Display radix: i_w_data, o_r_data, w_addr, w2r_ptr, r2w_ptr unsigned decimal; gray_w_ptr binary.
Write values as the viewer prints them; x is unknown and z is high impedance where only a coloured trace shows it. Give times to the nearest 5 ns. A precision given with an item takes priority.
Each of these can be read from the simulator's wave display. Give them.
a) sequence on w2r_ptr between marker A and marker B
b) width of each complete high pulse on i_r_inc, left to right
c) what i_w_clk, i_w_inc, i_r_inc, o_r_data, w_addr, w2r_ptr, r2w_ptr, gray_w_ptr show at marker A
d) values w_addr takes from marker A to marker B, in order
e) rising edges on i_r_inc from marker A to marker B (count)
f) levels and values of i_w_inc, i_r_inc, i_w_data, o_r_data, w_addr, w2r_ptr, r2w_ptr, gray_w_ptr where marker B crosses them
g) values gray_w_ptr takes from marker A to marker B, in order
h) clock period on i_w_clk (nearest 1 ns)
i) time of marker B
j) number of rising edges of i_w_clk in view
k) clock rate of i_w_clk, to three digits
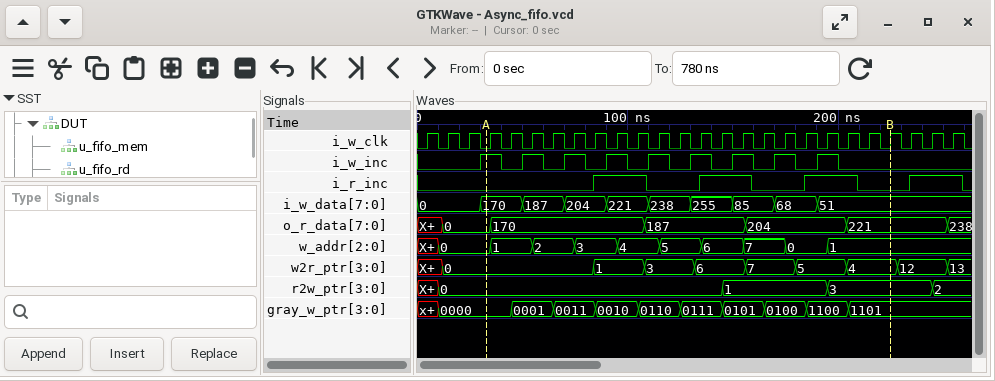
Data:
0, 1, 3, 6, 7, 5, 4
25 ns, 25 ns, 25 ns, 25 ns
i_w_clk=0, i_w_inc=1, i_r_inc=0, o_r_data=0, w_addr=0, w2r_ptr=0, r2w_ptr=0, gray_w_ptr=0000
0, 1, 2, 3, 4, 5, 6, 7, 0, 1
3
i_w_inc=0, i_r_inc=0, i_w_data=51, o_r_data=221, w_addr=1, w2r_ptr=4, r2w_ptr=3, gray_w_ptr=1101
0000, 0001, 0011, 0010, 0110, 0111, 0101, 0100, 1100, 1101
10 ns
225 ns
26
100 MHz
